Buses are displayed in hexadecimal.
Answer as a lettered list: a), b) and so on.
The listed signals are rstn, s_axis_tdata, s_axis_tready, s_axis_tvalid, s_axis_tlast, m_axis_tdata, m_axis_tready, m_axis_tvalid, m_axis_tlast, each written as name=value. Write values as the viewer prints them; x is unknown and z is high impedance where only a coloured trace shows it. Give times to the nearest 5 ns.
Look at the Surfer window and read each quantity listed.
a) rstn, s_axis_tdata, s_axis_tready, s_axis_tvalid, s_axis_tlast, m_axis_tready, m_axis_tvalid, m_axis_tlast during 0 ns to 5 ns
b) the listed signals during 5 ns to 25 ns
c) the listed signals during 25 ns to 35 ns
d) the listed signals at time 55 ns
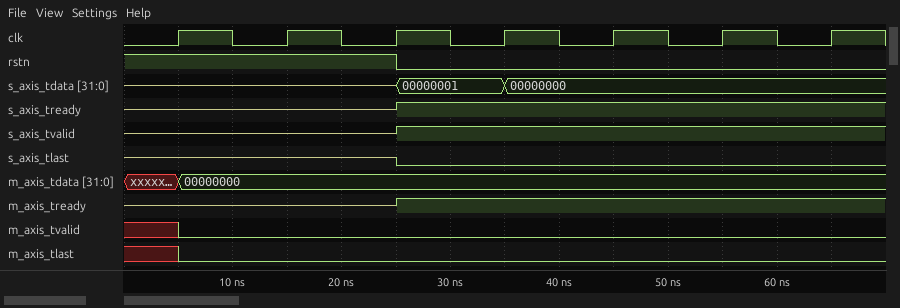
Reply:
a) rstn=1, s_axis_tdata=z, s_axis_tready=z, s_axis_tvalid=z, s_axis_tlast=z, m_axis_tready=z, m_axis_tvalid=x, m_axis_tlast=x
b) rstn=1, s_axis_tdata=z, s_axis_tready=z, s_axis_tvalid=z, s_axis_tlast=z, m_axis_tdata=00000000, m_axis_tready=z, m_axis_tvalid=0, m_axis_tlast=0
c) rstn=0, s_axis_tdata=00000001, s_axis_tready=1, s_axis_tvalid=1, s_axis_tlast=0, m_axis_tdata=00000000, m_axis_tready=1, m_axis_tvalid=0, m_axis_tlast=0
d) rstn=0, s_axis_tdata=00000000, s_axis_tready=1, s_axis_tvalid=1, s_axis_tlast=0, m_axis_tdata=00000000, m_axis_tready=1, m_axis_tvalid=0, m_axis_tlast=0
